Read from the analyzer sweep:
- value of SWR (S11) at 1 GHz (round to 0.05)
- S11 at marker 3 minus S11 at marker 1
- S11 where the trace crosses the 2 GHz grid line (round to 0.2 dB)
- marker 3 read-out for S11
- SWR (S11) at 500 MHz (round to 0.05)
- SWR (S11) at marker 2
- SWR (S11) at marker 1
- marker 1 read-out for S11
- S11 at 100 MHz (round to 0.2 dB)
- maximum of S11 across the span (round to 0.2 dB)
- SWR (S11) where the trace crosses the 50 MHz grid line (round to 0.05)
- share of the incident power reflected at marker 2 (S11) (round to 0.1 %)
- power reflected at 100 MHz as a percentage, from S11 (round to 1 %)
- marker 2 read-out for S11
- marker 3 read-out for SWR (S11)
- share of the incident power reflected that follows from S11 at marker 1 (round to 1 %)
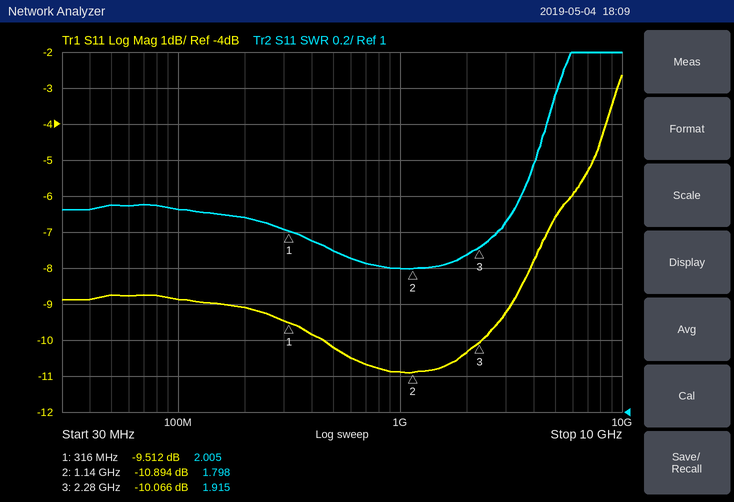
1.80
-0.554 dB
-10.4 dB
-10.066 dB
1.90
1.798
2.005
-9.512 dB
-8.8 dB
-2.6 dB
2.15
8.1 %
13 %
-10.894 dB
1.915
11 %
